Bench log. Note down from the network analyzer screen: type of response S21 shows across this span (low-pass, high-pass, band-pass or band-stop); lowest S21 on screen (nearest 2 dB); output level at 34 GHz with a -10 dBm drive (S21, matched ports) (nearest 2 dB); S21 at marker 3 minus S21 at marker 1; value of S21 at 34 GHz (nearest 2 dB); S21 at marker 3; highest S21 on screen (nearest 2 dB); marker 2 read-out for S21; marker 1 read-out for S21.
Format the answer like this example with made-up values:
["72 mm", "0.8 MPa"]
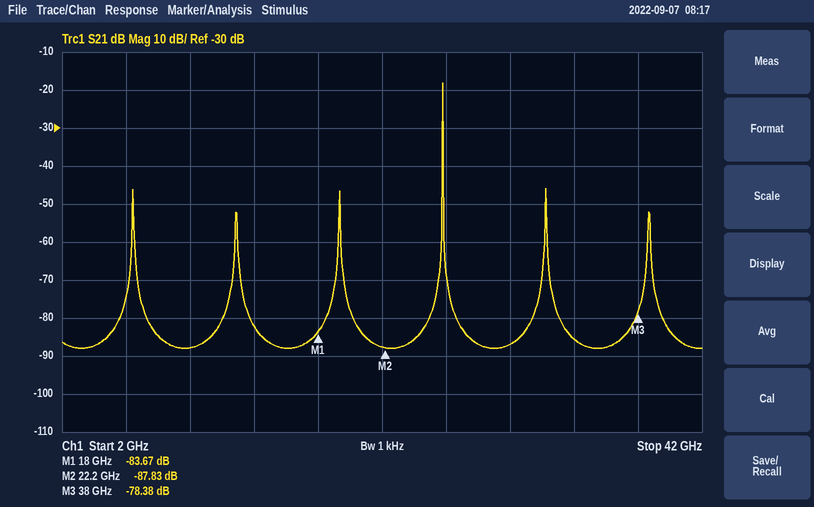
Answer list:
["band-pass", "-88 dB", "-96 dBm", "5.29 dB", "-86 dB", "-78.38 dB", "-18 dB", "-87.83 dB", "-83.67 dB"]
